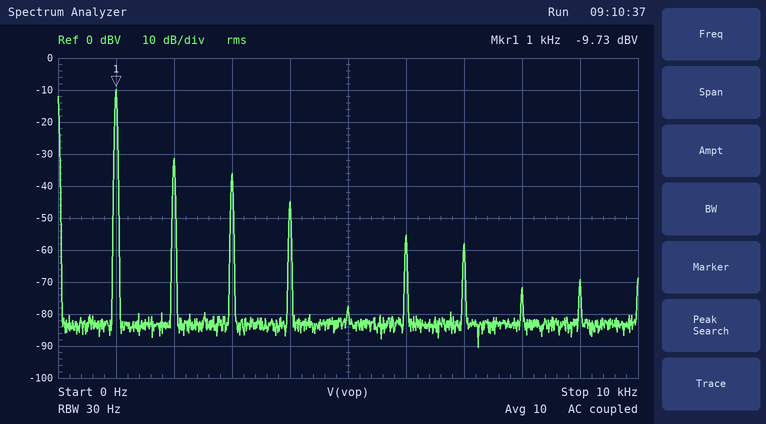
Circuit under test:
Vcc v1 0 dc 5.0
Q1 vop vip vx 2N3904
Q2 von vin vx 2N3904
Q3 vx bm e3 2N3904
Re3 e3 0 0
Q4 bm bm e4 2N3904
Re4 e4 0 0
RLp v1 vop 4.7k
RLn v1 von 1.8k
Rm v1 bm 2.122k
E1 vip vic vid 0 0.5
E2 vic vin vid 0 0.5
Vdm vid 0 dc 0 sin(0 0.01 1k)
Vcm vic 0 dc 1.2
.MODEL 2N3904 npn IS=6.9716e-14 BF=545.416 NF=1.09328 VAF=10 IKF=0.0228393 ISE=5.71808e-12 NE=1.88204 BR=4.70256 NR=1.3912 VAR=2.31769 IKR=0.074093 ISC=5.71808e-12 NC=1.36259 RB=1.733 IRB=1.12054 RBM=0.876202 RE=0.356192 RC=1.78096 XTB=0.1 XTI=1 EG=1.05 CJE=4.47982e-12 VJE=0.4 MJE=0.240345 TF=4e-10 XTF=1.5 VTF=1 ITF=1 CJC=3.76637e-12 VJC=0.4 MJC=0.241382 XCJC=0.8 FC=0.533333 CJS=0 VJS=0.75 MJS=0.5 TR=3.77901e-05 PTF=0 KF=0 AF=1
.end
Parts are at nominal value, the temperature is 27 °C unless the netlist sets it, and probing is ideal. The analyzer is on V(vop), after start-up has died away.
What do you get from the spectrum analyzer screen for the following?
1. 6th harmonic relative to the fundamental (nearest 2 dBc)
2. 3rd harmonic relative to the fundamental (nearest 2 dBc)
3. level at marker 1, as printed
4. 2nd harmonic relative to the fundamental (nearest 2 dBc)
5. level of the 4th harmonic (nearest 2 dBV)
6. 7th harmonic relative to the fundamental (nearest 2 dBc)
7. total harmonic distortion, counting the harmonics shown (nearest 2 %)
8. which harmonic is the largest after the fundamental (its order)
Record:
-46 dBc
-26 dBc
-9.73 dBV
-22 dBc
-44 dBV
-48 dBc
10 %
2
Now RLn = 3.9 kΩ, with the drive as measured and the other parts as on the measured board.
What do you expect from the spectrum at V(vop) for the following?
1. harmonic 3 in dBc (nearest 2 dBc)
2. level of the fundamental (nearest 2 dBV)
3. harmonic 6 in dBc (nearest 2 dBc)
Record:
-30 dBc
-16 dBV
-40 dBc
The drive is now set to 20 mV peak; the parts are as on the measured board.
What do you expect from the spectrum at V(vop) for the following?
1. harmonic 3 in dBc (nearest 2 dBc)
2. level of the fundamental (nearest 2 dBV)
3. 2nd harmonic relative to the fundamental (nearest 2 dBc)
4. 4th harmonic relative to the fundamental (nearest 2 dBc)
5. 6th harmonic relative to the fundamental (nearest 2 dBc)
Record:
-22 dBc
-6 dBV
-14 dBc
-40 dBc
-44 dBc
